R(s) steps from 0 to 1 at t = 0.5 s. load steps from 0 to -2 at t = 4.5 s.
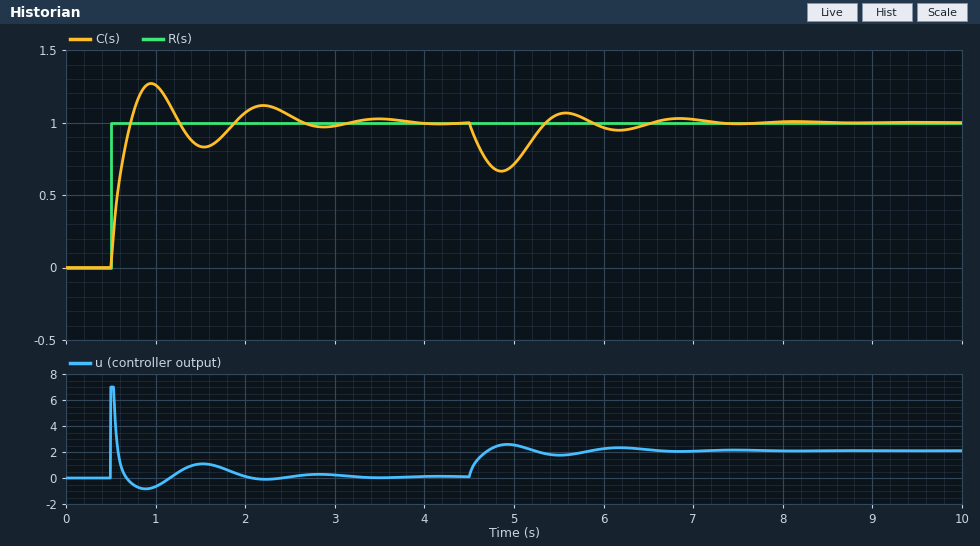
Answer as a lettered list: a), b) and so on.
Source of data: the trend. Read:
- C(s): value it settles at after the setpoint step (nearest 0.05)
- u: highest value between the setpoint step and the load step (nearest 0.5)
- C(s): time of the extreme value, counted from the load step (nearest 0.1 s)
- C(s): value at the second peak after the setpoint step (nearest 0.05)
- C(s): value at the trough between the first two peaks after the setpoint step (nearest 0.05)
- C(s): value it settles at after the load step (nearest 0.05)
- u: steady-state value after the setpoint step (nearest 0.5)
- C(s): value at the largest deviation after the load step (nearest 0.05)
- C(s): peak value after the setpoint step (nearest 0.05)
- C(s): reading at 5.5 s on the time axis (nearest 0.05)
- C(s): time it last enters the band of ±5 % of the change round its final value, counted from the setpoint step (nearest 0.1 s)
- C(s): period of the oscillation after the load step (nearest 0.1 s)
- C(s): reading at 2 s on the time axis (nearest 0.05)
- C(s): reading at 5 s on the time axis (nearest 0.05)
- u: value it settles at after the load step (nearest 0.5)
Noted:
a) 1.00
b) 7.0
c) 0.4 s
d) 1.10
e) 0.85
f) 1.00
g) 0.0
h) 0.65
i) 1.25
j) 1.05
k) 2.0 s
l) 1.3 s
m) 1.05
n) 0.70
o) 2.0
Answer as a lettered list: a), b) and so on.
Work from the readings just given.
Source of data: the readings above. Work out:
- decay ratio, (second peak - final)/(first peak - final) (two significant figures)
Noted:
a) 0.40
